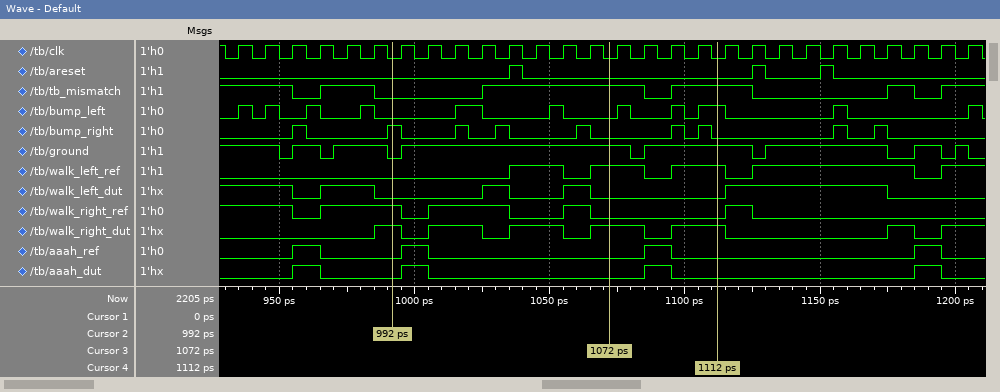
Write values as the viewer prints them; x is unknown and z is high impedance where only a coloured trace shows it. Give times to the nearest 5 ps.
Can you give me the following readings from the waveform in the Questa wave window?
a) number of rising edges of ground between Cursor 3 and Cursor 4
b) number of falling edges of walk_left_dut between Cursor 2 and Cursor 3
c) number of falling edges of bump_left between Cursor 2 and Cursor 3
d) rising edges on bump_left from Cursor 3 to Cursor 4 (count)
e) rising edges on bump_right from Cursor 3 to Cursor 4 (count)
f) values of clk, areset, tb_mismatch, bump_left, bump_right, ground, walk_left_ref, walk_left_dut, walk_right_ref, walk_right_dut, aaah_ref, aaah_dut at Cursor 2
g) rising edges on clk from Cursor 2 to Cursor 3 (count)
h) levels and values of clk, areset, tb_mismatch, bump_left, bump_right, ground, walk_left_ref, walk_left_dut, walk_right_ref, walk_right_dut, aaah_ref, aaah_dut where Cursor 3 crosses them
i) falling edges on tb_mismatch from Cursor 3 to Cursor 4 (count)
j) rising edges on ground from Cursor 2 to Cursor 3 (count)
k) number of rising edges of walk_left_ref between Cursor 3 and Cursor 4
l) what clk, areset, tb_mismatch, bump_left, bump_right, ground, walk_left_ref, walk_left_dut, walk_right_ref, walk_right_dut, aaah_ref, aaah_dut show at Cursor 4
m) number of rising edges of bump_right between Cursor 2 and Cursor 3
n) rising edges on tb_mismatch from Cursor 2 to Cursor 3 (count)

1
2
2
3
2
clk=0, areset=0, tb_mismatch=0, bump_left=0, bump_right=1, ground=0, walk_left_ref=0, walk_left_dut=0, walk_right_ref=1, walk_right_dut=1, aaah_ref=0, aaah_dut=0
8
clk=0, areset=0, tb_mismatch=1, bump_left=0, bump_right=0, ground=1, walk_left_ref=1, walk_left_dut=0, walk_right_ref=0, walk_right_dut=1, aaah_ref=0, aaah_dut=0
1
1
1
clk=0, areset=0, tb_mismatch=1, bump_left=1, bump_right=0, ground=1, walk_left_ref=1, walk_left_dut=0, walk_right_ref=0, walk_right_dut=1, aaah_ref=0, aaah_dut=0
3
1
